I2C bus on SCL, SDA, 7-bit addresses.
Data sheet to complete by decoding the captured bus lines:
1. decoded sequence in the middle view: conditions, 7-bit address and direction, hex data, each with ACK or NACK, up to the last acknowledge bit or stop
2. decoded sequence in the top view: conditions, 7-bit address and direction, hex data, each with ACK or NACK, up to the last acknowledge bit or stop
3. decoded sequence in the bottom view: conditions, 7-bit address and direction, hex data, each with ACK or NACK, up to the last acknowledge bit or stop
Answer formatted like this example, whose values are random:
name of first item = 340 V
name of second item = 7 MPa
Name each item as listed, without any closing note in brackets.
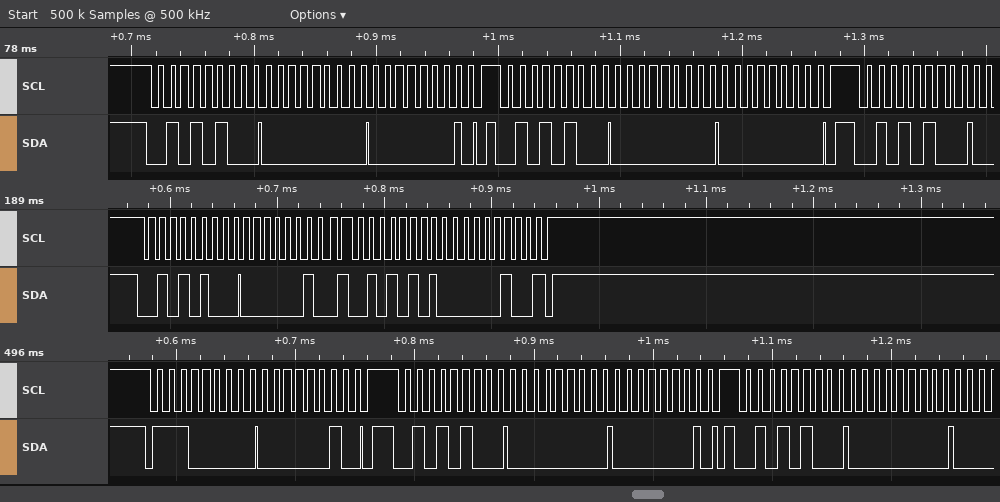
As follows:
decoded sequence in the middle view: conditions, 7-bit address and direction, hex data, each with ACK or NACK, up to the last acknowledge bit or stop = start, address 2A write ACK, 02 ACK, repeated start, address 2A read ACK, 04 NACK, stop
decoded sequence in the top view: conditions, 7-bit address and direction, hex data, each with ACK or NACK, up to the last acknowledge bit or stop = start, address 2A write ACK, 00 ACK, 01 ACK, stop, start, address 2A write ACK, 00 ACK, 00 ACK, stop, start, address 2A write ACK
decoded sequence in the bottom view: conditions, 7-bit address and direction, hex data, each with ACK or NACK, up to the last acknowledge bit or stop = start, address 70 write ACK, 02 ACK, stop, start, address 2A write ACK, 00 ACK, 01 ACK, stop, start, address 2A write ACK, 00 ACK
